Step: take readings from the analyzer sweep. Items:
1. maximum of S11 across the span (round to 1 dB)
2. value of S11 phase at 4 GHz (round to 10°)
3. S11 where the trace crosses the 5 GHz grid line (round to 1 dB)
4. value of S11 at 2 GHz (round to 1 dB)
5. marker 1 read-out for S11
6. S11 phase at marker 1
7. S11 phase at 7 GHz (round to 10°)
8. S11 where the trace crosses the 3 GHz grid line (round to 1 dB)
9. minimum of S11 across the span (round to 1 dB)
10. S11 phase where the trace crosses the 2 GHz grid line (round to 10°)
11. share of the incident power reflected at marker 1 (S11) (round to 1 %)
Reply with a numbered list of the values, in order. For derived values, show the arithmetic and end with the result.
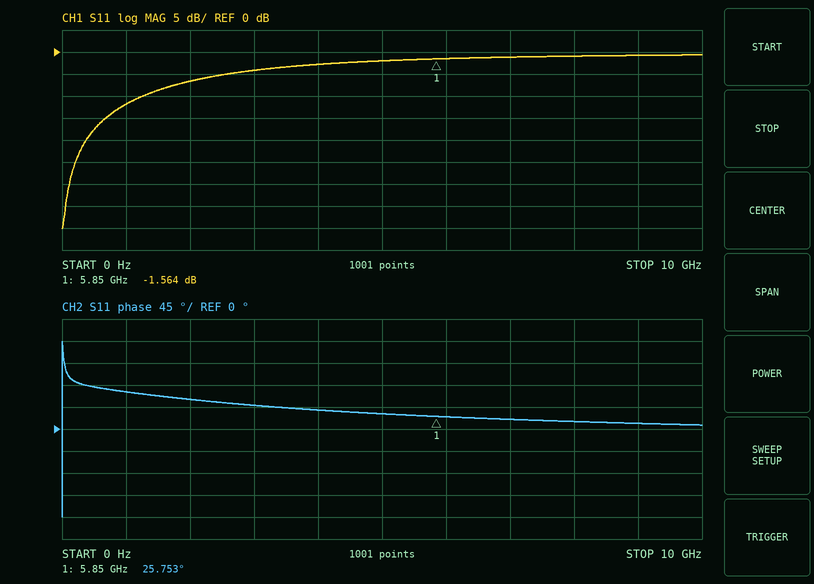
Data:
1. -1 dB
2. 40°
3. -2 dB
4. -7 dB
5. -1.564 dB
6. 25.753°
7. 20°
8. -4 dB
9. -40 dB
10. 60°
11. 10^(-1.564/10) ≈ 70 %
